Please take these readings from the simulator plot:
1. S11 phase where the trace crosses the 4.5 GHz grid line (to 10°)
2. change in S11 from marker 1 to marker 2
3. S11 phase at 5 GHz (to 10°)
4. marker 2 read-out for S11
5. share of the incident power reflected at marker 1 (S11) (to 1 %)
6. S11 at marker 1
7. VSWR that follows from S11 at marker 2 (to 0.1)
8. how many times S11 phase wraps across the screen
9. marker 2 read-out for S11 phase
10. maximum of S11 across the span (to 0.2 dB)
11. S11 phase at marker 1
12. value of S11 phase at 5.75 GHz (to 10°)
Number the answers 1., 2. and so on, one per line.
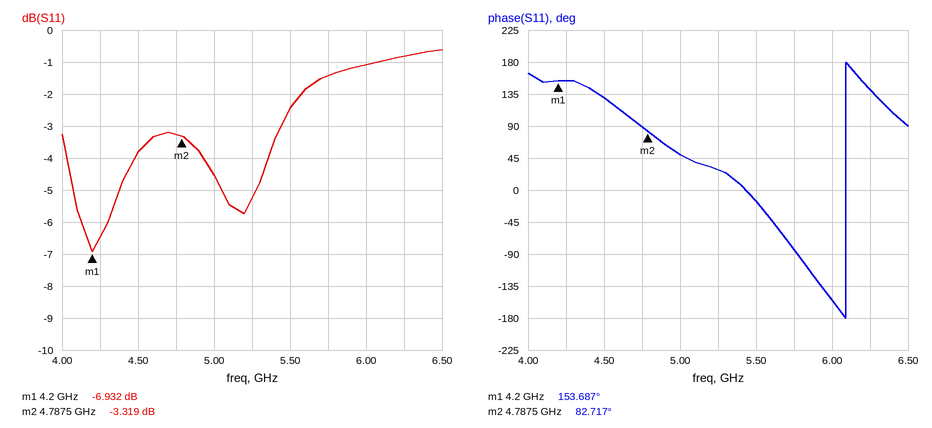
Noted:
1. 130°
2. 3.613 dB
3. 50°
4. -3.319 dB
5. 20 %
6. -6.932 dB
7. 5.3
8. 1
9. 82.717°
10. -0.6 dB
11. 153.687°
12. -80°
